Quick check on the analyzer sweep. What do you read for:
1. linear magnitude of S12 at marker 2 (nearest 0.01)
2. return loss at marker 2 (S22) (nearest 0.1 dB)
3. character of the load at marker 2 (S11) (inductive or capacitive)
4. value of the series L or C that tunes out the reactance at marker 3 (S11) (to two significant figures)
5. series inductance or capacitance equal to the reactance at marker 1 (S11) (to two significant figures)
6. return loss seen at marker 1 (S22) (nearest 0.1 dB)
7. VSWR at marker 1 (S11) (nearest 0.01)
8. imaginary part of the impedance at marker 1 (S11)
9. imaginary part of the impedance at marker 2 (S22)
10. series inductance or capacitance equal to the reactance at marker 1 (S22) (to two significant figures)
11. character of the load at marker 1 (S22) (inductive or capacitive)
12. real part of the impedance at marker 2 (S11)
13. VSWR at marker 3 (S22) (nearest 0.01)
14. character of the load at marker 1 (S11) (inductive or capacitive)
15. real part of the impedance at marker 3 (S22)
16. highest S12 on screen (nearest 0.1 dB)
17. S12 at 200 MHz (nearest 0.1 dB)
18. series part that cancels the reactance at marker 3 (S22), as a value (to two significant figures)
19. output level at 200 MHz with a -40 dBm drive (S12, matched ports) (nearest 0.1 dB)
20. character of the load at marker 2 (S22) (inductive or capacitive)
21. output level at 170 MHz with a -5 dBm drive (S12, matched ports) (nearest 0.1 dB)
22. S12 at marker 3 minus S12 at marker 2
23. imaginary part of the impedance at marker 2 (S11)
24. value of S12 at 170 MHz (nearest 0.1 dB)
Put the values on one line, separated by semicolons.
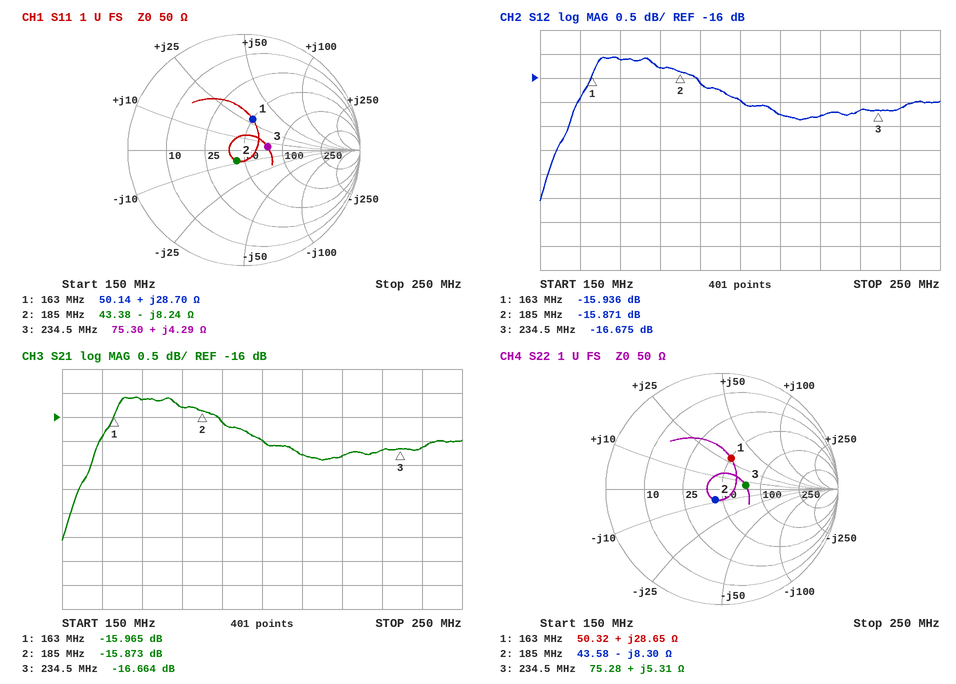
0.16; 19.0 dB; capacitive; 160 pF; 28 nH; 11.2 dB; 1.76; +28.70 Ω; -8.30 Ω; 28 nH; inductive; 43.38 Ω; 1.52; inductive; 75.28 Ω; -15.6 dB; -16.5 dB; 130 pF; -56.5 dBm; capacitive; -20.6 dBm; -0.804 dB; -8.24 Ω; -15.6 dB
